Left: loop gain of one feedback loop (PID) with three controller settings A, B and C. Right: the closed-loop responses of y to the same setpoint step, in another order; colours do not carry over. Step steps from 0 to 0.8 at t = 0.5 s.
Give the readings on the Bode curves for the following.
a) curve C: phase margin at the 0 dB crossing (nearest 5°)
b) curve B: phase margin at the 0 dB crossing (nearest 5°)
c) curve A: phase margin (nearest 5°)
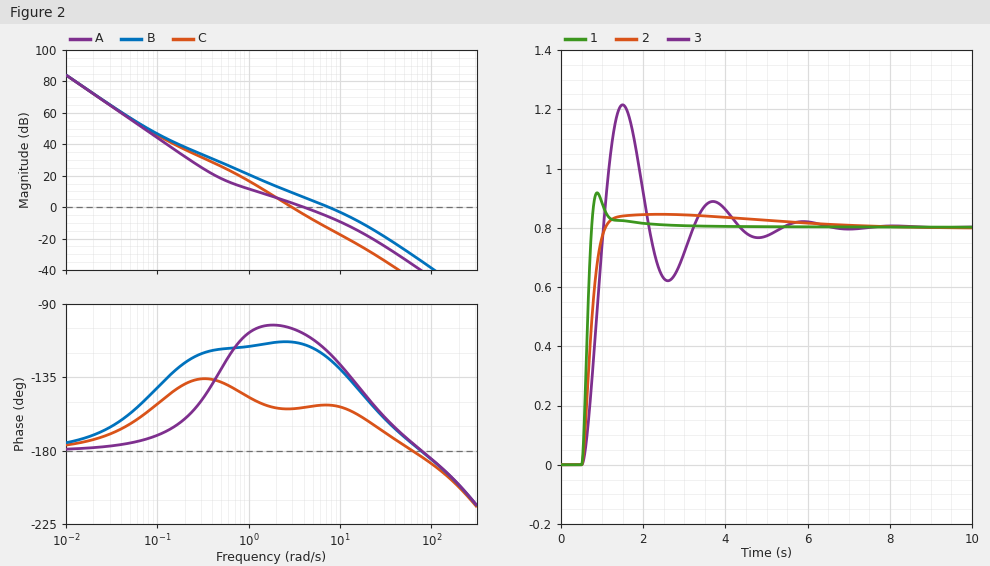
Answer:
25°
55°
70°
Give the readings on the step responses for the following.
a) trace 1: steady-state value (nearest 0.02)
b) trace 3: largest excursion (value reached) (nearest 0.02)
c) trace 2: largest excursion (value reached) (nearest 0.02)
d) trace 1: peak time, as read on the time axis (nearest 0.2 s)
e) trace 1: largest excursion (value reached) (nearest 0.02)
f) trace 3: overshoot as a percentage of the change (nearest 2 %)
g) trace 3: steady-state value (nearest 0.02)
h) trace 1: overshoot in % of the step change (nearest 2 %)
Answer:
0.80
1.22
0.84
0.8 s
0.92
52 %
0.80
14 %
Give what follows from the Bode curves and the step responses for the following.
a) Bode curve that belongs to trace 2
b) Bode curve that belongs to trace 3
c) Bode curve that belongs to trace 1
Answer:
A
C
B
